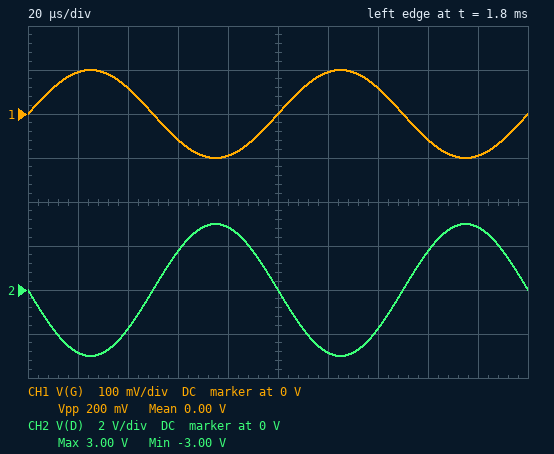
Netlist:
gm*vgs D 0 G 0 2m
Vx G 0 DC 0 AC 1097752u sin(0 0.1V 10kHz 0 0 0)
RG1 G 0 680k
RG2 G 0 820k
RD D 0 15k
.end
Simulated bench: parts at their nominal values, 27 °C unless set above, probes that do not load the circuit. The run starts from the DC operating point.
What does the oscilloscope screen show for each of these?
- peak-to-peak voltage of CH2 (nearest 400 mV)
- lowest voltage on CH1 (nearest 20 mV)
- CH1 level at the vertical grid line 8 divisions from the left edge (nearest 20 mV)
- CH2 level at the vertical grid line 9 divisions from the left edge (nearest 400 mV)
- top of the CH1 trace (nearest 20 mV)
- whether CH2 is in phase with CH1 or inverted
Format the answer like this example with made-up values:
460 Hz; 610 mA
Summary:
6.0 V; -100 mV; -60 mV; 2.8 V; 100 mV; inverted
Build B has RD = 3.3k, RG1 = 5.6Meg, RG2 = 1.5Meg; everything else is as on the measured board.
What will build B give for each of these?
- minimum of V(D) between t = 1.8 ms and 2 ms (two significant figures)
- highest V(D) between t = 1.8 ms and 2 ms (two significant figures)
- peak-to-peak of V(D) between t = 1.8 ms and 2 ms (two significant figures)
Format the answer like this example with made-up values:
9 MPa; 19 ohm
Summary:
-660 mV; 660 mV; 1.3 V
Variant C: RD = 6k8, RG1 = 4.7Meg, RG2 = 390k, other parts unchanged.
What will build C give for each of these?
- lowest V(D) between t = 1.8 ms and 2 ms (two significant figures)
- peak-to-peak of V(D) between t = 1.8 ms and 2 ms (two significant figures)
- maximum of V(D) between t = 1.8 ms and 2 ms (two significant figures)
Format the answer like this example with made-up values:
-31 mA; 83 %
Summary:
-1.4 V; 2.7 V; 1.4 V
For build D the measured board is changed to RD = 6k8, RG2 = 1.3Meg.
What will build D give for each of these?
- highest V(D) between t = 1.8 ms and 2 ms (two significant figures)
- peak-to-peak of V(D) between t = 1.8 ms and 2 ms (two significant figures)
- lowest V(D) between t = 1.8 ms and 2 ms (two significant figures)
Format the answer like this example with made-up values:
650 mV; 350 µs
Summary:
1.4 V; 2.7 V; -1.4 V
